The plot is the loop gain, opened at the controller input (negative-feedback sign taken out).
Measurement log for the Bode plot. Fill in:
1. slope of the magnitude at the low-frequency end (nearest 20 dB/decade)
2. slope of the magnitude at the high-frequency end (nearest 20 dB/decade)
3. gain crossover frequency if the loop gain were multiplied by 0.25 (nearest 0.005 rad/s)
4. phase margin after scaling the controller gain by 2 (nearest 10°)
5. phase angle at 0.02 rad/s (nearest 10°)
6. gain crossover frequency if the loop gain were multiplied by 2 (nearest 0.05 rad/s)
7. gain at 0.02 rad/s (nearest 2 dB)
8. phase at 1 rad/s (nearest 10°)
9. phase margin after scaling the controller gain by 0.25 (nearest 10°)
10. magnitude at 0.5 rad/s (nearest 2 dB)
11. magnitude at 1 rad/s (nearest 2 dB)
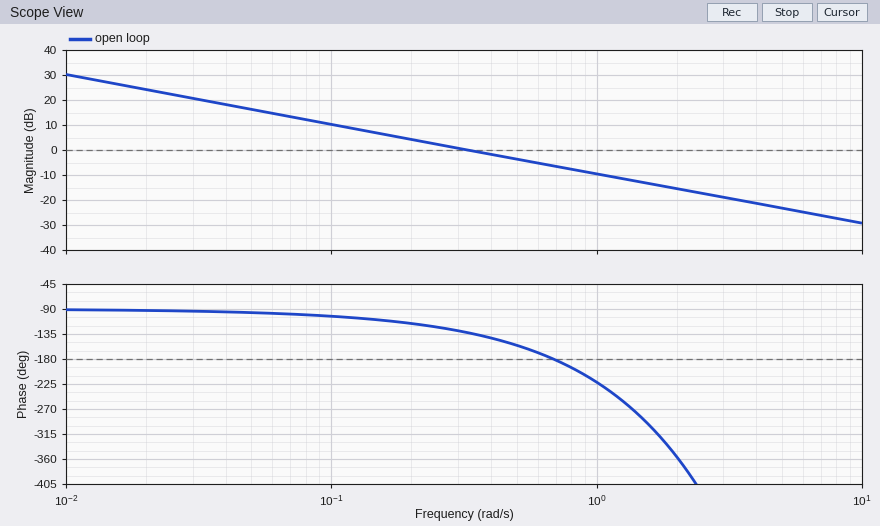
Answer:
-20 dB/decade
-20 dB/decade
0.080 rad/s
0°
-90°
0.65 rad/s
24 dB
-220°
80°
-4 dB
-10 dB
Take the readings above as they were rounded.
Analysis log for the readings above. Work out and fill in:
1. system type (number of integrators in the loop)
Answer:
1
